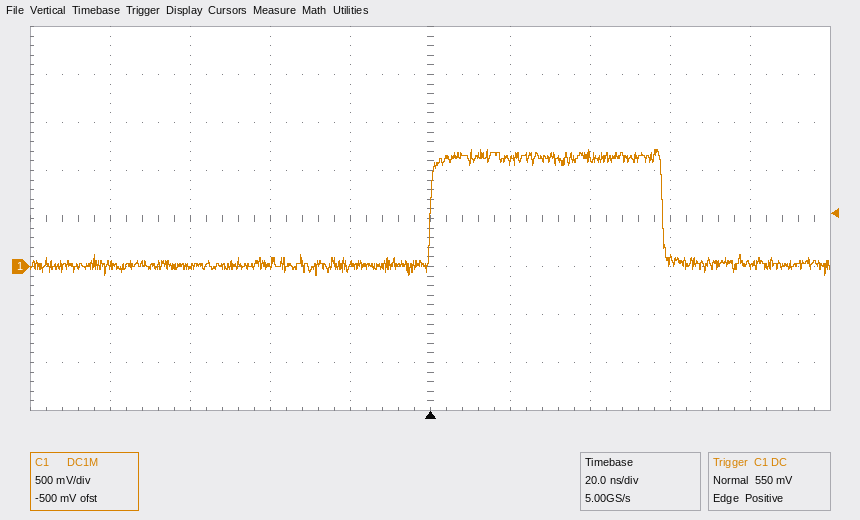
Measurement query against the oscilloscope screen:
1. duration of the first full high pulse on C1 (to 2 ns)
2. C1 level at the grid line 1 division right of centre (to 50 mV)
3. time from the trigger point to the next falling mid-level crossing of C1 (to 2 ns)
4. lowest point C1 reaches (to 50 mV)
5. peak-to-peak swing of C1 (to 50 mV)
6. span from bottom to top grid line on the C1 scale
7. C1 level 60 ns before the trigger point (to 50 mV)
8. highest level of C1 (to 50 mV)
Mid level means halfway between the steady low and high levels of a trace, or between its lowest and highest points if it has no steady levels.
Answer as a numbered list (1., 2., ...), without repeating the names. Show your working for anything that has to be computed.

1. 58 ns
2. 1.10 V
3. 58 ns
4. -100 mV
5. 1.20 V − (-100 mV) = 1.30 V
6. 4 V
7. 0 mV
8. 1.20 V
